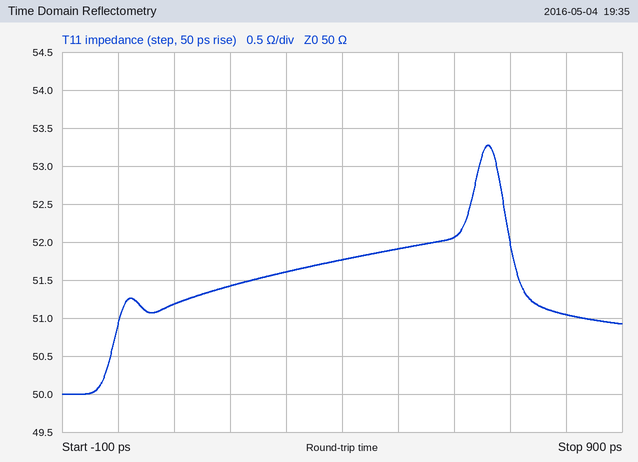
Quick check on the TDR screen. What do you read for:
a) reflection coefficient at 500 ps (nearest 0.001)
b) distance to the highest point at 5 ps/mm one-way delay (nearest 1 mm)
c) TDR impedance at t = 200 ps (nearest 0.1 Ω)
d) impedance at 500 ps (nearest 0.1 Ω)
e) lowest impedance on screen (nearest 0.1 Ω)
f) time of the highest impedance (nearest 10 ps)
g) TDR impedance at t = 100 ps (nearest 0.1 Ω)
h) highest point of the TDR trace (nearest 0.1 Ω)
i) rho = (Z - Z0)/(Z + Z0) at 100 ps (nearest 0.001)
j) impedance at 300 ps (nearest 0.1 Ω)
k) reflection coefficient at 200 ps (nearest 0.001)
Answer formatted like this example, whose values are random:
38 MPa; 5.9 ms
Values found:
+0.019; 66 mm; 51.4 Ω; 51.9 Ω; 50.0 Ω; 660 ps; 51.2 Ω; 53.3 Ω; +0.012; 51.6 Ω; +0.014
